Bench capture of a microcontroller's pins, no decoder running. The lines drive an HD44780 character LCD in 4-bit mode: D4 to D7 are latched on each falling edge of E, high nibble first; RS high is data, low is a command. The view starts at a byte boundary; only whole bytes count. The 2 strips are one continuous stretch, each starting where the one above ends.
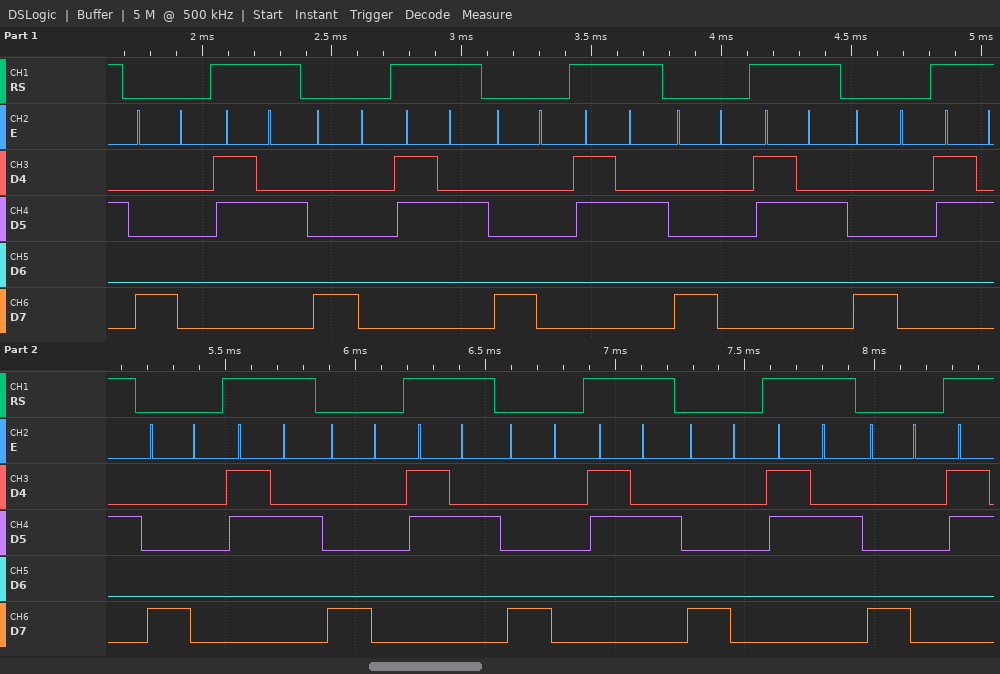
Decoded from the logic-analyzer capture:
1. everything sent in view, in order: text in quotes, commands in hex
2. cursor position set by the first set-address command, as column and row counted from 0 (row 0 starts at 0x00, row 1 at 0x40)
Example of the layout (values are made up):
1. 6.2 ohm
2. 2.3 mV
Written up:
1. 0x80 "2" 0x80 "2" 0x80 "2" 0x80 "2" 0x80 "2" 0x80 "2" 0x80 "2" 0x80 "2" 0x80 "2" 0x80
2. column 0, row 0
